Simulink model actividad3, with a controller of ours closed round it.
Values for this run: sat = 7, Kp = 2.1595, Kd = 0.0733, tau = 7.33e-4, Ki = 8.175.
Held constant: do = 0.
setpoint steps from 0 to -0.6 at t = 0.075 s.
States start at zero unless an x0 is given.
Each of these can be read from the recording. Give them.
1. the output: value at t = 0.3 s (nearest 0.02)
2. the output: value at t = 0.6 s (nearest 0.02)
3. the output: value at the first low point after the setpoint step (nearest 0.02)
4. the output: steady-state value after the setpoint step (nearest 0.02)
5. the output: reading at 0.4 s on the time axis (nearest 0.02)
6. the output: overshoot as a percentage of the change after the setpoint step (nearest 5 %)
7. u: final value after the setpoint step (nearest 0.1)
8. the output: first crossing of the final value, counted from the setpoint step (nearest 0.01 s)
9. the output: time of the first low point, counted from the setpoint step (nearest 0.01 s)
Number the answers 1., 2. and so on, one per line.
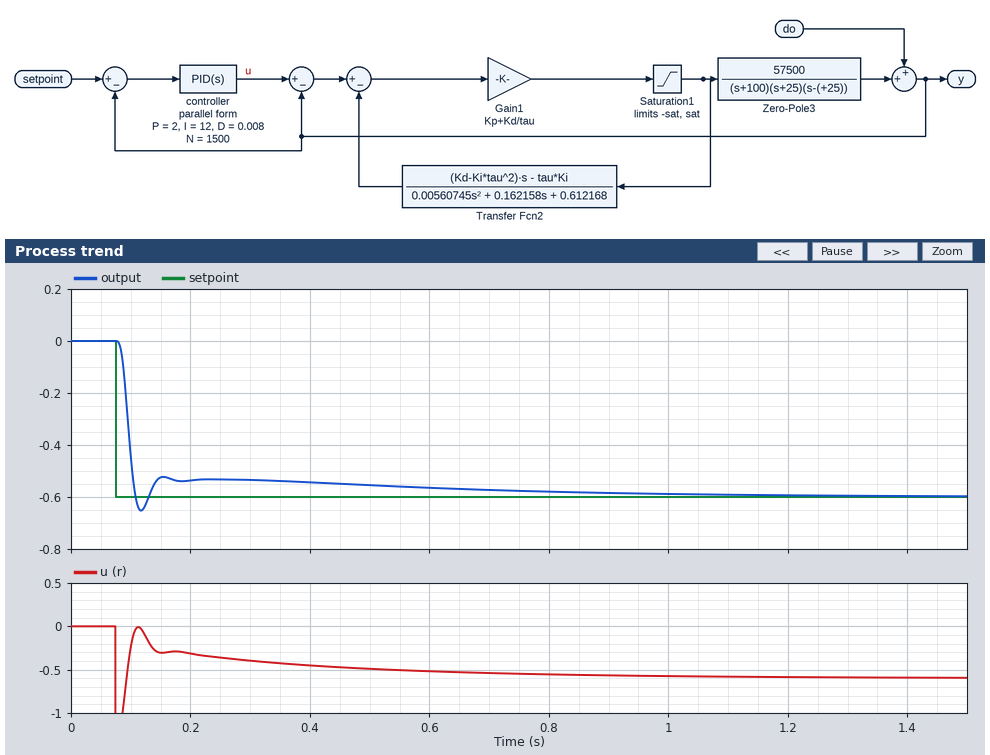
1. -0.54
2. -0.56
3. -0.66
4. -0.60
5. -0.54
6. 10 %
7. -0.6
8. 0.03 s
9. 0.04 s
